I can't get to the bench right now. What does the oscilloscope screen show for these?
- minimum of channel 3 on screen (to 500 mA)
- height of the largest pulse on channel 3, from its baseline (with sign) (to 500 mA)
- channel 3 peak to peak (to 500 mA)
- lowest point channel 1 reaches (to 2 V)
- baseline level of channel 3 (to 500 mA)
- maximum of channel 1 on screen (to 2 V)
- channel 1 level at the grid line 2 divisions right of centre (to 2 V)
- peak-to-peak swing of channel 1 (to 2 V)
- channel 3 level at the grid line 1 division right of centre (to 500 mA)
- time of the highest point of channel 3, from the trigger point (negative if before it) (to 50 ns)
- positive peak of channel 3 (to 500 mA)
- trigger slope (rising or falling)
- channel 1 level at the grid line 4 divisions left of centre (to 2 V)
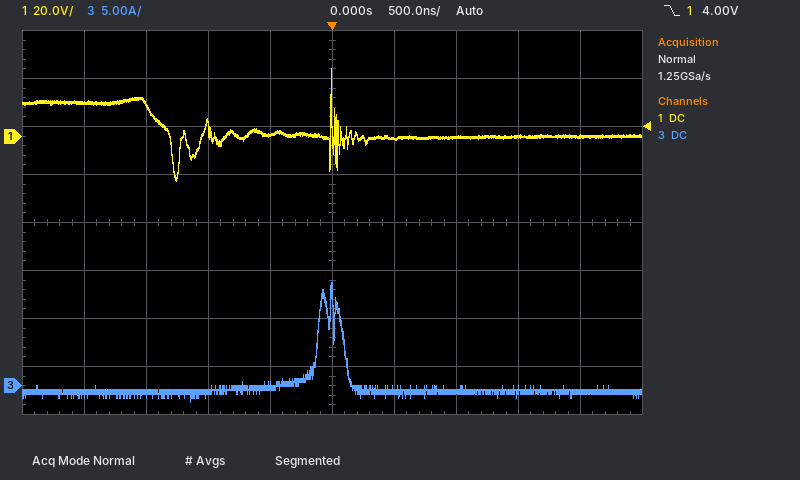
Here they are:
-1.5 A
+11.5 A
12.5 A
-18 V
-500 mA
28 V
0 V
46 V
-500 mA
0 ns
11.0 A
falling
14 V
